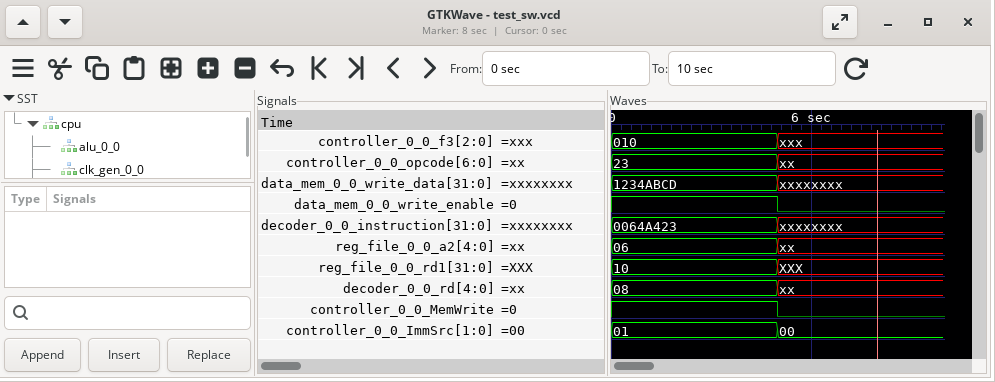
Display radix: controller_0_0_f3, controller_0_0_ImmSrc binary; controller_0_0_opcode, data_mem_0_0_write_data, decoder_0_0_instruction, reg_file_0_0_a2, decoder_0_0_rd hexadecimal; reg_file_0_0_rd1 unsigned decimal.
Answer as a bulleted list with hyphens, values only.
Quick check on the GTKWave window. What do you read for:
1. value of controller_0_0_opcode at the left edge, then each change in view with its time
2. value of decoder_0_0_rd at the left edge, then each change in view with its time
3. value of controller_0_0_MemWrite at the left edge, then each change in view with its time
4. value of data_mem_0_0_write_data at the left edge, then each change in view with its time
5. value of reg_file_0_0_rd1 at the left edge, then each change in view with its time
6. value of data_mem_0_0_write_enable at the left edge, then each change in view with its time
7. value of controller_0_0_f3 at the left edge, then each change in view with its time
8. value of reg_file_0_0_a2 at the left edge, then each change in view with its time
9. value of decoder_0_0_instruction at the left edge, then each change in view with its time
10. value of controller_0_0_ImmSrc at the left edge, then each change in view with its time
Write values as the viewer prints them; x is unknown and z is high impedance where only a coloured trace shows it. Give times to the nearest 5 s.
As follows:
- 23, xx at 5 s
- 08, xx at 5 s
- 1, 0 at 5 s
- 1234ABCD, xxxxxxxx at 5 s
- 10, XXX at 5 s
- 1, 0 at 5 s
- 010, xxx at 5 s
- 06, xx at 5 s
- 0064A423, xxxxxxxx at 5 s
- 01, 00 at 5 s
